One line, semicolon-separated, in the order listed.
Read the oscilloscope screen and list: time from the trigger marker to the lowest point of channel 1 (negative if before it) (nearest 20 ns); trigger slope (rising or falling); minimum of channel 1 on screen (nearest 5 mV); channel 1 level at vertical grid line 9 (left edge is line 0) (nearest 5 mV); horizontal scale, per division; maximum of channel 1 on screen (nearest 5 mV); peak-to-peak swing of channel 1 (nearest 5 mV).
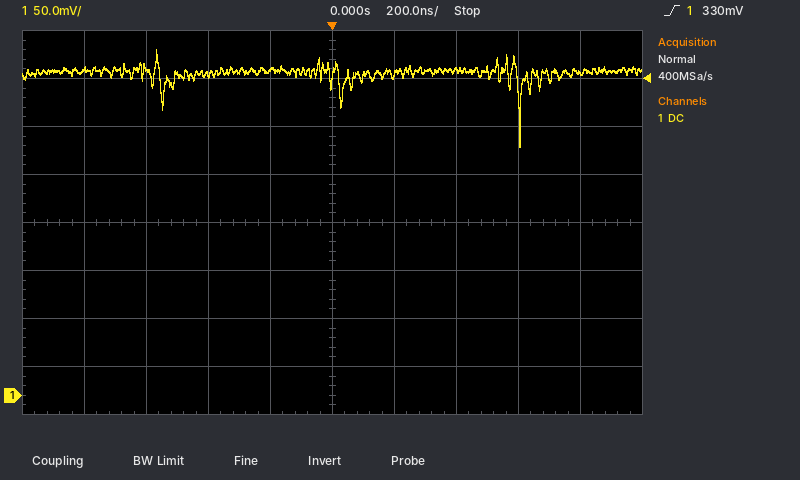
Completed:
+600 ns; rising; 260 mV; 335 mV; 200 ns; 360 mV; 100 mV
